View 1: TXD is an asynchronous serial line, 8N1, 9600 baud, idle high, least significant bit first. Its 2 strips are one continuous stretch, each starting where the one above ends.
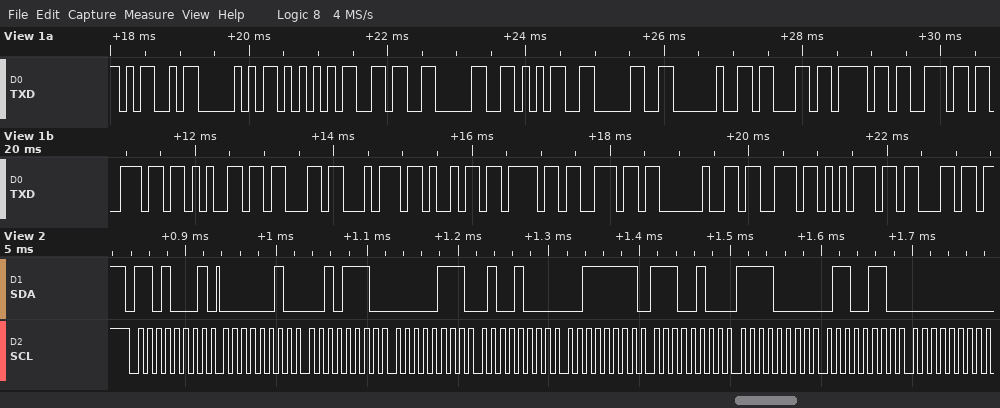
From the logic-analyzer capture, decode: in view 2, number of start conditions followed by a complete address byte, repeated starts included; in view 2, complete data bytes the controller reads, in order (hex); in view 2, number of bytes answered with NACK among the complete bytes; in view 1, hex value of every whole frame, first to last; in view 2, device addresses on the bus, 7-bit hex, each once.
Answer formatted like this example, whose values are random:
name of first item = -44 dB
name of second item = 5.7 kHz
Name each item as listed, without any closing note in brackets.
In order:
in view 2, number of start conditions followed by a complete address byte, repeated starts included = 1
in view 2, complete data bytes the controller reads, in order = 02 2E 07 48 3F E4 F0 66 00
in view 2, number of bytes answered with NACK among the complete bytes = 0
in view 1, hex value of every whole frame, first to last = 0x4D 0x50 0x55 0x36 0x30 0x35 0x30 0x20 0x63 0x6F 0x6E 0x6E 0x65 0x63 0x74 0x69 0x6F 0x6E 0x20 0x73 0x75 0x63
in view 2, device addresses on the bus, 7-bit hex, each once = 0x68
